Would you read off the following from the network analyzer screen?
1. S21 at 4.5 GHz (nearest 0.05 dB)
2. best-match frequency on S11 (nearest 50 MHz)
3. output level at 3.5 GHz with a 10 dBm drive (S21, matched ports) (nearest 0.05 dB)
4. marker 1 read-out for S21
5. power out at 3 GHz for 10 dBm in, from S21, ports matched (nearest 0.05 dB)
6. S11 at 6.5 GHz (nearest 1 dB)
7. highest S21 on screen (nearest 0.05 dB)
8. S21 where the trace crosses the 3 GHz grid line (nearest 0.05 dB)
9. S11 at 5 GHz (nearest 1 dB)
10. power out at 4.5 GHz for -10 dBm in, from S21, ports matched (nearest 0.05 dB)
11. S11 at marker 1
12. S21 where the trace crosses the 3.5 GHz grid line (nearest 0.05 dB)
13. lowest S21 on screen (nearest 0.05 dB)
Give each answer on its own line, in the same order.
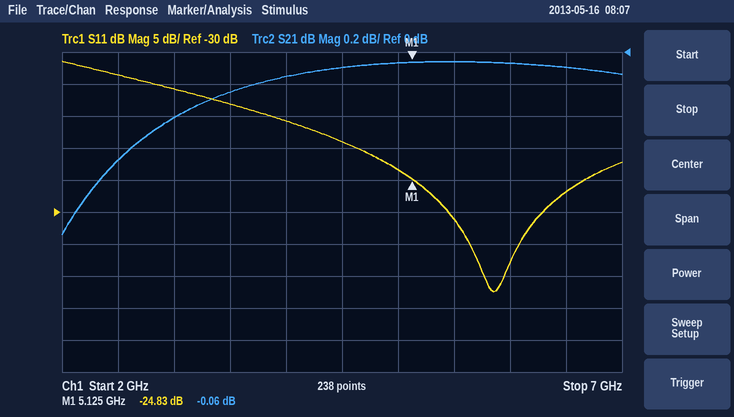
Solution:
-0.10 dB
5.85 GHz
9.75 dBm
-0.06 dB
9.60 dBm
-27 dB
-0.05 dB
-0.40 dB
-23 dB
-10.10 dBm
-24.83 dB
-0.25 dB
-1.15 dB
